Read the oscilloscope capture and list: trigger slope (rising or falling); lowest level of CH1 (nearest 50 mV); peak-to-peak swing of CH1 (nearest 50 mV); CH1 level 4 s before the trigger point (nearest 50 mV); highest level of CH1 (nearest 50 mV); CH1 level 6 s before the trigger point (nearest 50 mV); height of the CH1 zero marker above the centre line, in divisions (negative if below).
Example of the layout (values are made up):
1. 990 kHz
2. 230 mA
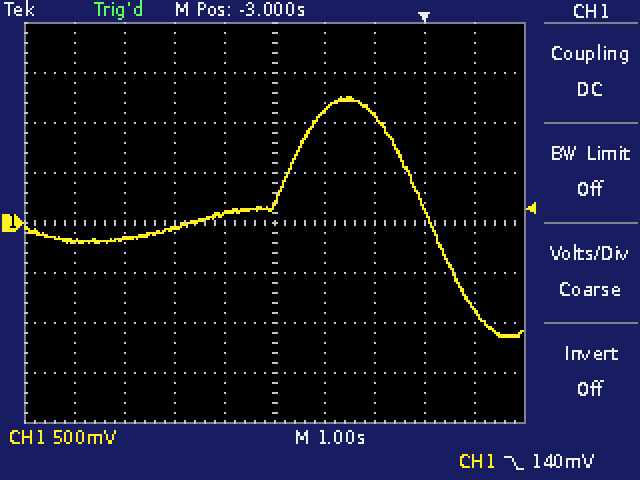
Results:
1. falling
2. -1.15 V
3. 2.40 V
4. 100 mV
5. 1.25 V
6. -150 mV
7. 0.0 div
